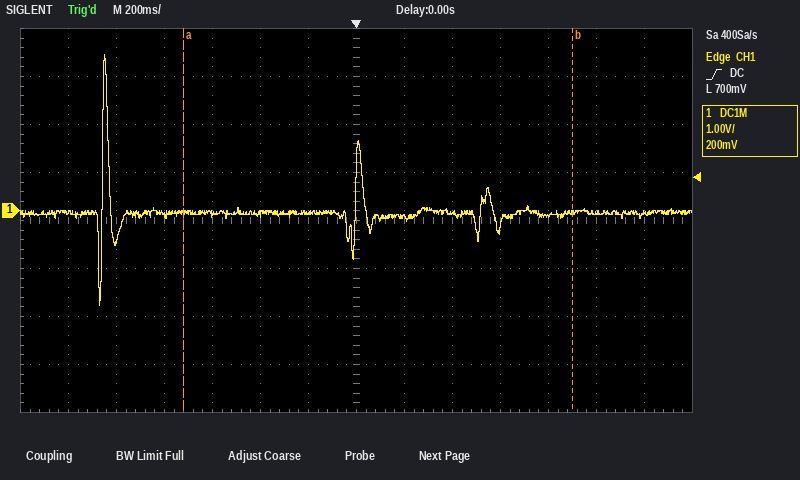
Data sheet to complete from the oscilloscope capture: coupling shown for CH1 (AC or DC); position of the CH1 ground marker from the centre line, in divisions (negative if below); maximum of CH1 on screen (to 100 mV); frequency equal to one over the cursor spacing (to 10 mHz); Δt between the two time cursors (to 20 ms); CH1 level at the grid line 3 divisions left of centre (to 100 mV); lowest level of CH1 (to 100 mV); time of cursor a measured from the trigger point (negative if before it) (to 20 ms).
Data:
DC
+0.2 div
3.3 V
620 mHz
1.62 s
-100 mV
-2.0 V
-720 ms
